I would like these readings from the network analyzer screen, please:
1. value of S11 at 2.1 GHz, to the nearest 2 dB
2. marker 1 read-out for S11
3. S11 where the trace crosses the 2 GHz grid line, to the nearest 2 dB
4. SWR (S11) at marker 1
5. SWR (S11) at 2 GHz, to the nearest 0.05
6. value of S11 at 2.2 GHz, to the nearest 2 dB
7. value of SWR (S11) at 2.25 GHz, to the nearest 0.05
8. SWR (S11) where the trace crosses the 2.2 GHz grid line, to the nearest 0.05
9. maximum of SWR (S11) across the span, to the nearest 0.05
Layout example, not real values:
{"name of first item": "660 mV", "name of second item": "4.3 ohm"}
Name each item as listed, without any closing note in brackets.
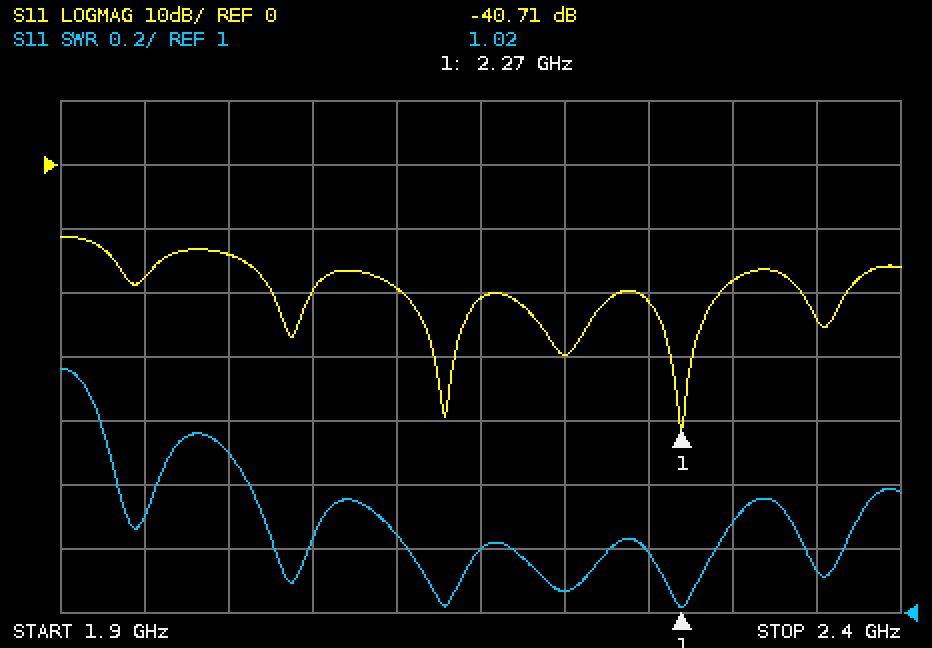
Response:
{"value of S11 at 2.1 GHz, to the nearest 2 dB": "-20 dB", "marker 1 read-out for S11": "-40.71 dB", "S11 where the trace crosses the 2 GHz grid line, to the nearest 2 dB": "-14 dB", "SWR (S11) at marker 1": "1.02", "SWR (S11) at 2 GHz, to the nearest 0.05": "1.50", "value of S11 at 2.2 GHz, to the nearest 2 dB": "-30 dB", "value of SWR (S11) at 2.25 GHz, to the nearest 0.05": "1.20", "SWR (S11) where the trace crosses the 2.2 GHz grid line, to the nearest 0.05": "1.05", "maximum of SWR (S11) across the span, to the nearest 0.05": "1.75"}
